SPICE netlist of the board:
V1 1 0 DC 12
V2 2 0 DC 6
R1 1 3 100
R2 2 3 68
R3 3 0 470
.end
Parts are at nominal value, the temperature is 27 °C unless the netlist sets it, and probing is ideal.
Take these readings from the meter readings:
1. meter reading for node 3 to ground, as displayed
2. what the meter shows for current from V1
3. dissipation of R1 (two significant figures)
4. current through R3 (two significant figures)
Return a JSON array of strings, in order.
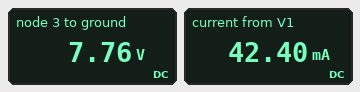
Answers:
["7.76 V", "42.40 mA", "180 mW", "17 mA"]
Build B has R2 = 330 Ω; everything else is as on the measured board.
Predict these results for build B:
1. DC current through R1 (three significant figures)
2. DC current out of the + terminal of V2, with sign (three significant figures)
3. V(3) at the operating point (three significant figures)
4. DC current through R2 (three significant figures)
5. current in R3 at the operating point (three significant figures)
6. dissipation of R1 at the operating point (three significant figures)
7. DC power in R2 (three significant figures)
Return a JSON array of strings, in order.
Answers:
["28.8 mA", "-9.44 mA", "9.12 V", "9.44 mA", "19.4 mA", "83.2 mW", "29.4 mW"]
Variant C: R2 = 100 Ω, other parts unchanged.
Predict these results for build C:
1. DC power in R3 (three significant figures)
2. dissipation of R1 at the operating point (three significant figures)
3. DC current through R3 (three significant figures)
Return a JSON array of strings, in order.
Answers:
["141 mW", "149 mW", "17.3 mA"]
